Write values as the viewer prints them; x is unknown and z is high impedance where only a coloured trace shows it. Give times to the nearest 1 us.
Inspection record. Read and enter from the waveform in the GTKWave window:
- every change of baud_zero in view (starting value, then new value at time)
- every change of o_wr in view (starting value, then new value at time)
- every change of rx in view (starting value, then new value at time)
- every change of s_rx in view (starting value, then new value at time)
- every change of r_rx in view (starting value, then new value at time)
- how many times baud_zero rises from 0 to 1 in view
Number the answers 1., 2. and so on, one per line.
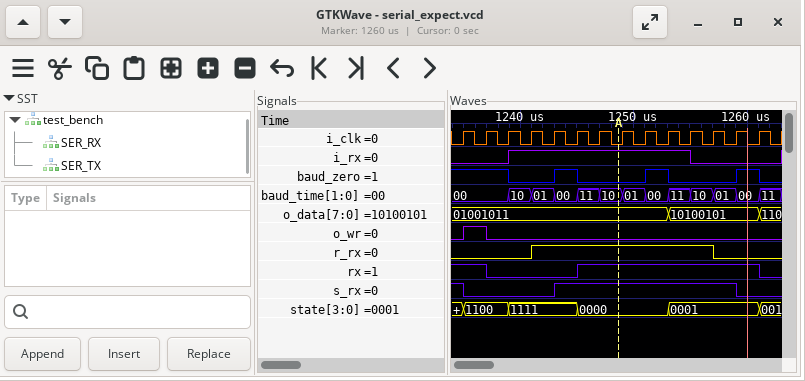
1. 1, 0 at 1239 us, 1 at 1243 us, 0 at 1245 us, 1 at 1251 us, 0 at 1253 us, 1 at 1259 us, 0 at 1261 us
2. 0, 1 at 1235 us, 0 at 1237 us
3. 1, 0 at 1237 us, 1 at 1245 us, 0 at 1261 us
4. 1, 0 at 1235 us, 1 at 1243 us, 0 at 1259 us
5. 0, 1 at 1241 us, 0 at 1257 us
6. 3
